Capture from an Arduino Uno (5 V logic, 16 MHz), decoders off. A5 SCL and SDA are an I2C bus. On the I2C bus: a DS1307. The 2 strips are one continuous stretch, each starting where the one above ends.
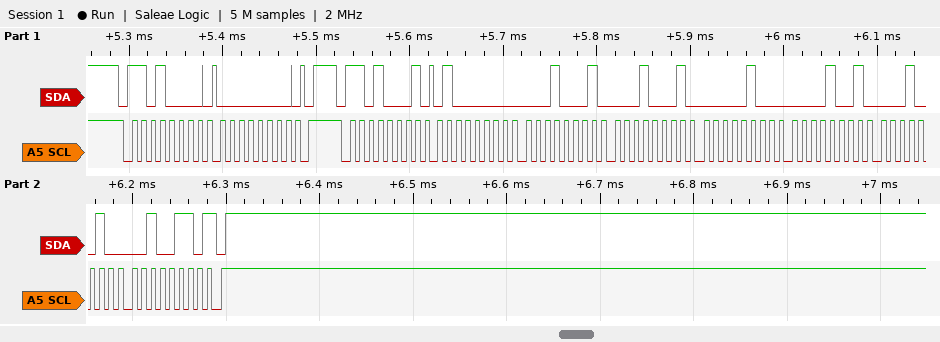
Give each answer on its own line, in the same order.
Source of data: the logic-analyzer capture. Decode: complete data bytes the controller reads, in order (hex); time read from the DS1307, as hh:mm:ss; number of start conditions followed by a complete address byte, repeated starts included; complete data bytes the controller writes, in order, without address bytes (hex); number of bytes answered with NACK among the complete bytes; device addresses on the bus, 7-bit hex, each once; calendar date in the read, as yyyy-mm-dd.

40 11 11 04 09 12 26
11:11:40
2
00
1
0x68
2026-12-09
